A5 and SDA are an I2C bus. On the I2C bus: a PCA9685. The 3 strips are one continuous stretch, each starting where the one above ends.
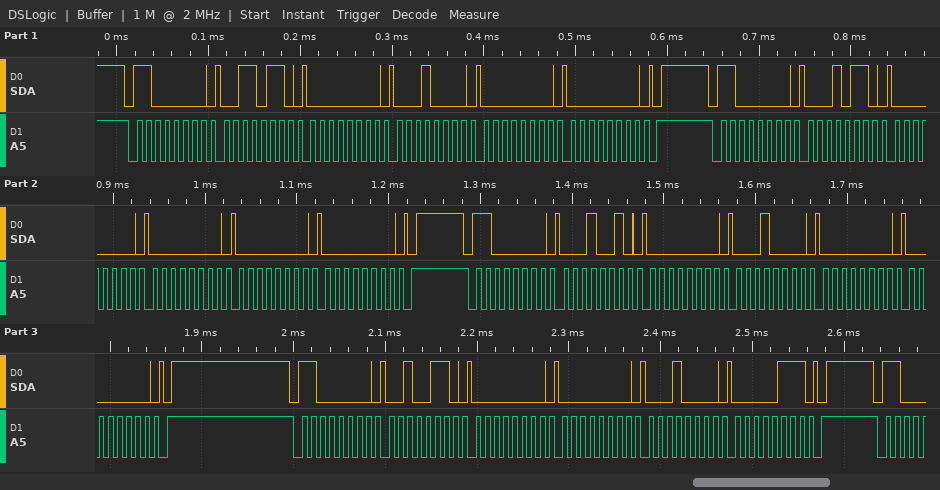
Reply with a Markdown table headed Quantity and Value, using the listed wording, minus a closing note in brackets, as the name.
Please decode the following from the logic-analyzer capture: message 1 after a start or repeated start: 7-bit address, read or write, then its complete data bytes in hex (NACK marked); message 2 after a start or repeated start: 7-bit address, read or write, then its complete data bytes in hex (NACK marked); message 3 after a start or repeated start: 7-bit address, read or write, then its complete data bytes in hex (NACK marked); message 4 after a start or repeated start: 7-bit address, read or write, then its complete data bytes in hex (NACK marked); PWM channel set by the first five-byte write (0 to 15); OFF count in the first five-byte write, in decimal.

| Quantity | Value |
|---|---|
| message 1 after a start or repeated start: 7-bit address, read or write, then its complete data bytes in hex | 0x60 write: 36 00 10 00 00 |
| message 2 after a start or repeated start: 7-bit address, read or write, then its complete data bytes in hex | 0x60 write: 16 00 00 00 00 |
| message 3 after a start or repeated start: 7-bit address, read or write, then its complete data bytes in hex | 0x60 write: 12 00 10 00 00 |
| message 4 after a start or repeated start: 7-bit address, read or write, then its complete data bytes in hex | 0x60 write: 26 00 00 10 07 |
| PWM channel set by the first five-byte write | 12 |
| OFF count in the first five-byte write, in decimal | 0 |
